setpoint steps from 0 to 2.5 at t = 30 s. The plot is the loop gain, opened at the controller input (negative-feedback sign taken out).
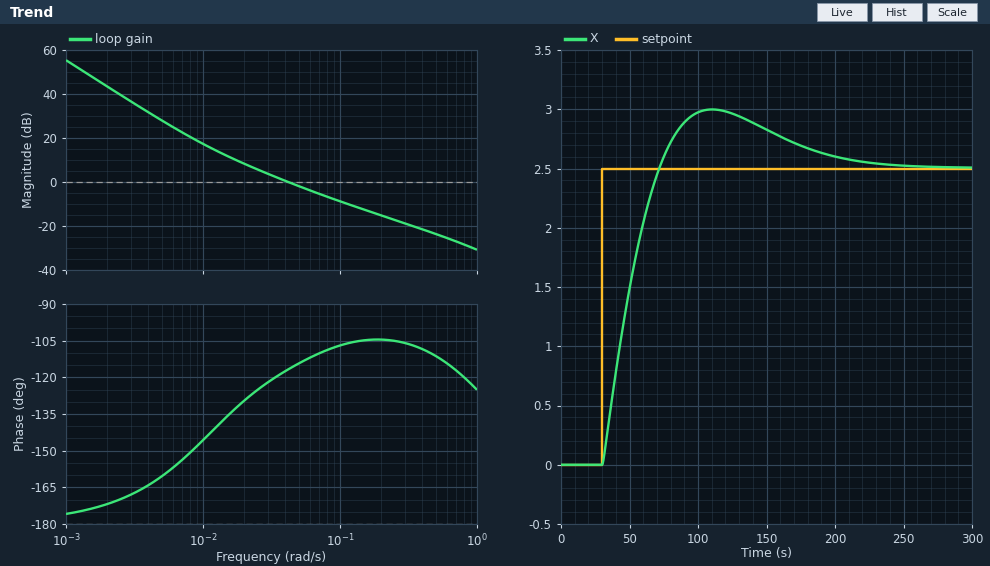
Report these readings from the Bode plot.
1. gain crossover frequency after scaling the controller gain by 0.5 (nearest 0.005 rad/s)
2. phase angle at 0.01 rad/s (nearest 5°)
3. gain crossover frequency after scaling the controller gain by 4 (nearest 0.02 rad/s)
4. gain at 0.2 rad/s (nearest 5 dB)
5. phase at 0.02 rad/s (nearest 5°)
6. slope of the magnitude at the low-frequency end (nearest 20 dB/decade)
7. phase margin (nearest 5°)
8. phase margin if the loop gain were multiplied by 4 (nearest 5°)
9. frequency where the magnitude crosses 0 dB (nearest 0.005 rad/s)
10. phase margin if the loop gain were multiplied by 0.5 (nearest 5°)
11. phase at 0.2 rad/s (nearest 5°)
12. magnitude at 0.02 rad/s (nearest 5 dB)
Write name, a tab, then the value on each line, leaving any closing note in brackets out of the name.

gain crossover frequency after scaling the controller gain by 0.5	0.025 rad/s
phase angle at 0.01 rad/s	-145°
gain crossover frequency after scaling the controller gain by 4	0.14 rad/s
gain at 0.2 rad/s	-15 dB
phase at 0.02 rad/s	-130°
slope of the magnitude at the low-frequency end	-40 dB/decade
phase margin	65°
phase margin if the loop gain were multiplied by 4	75°
frequency where the magnitude crosses 0 dB	0.040 rad/s
phase margin if the loop gain were multiplied by 0.5	55°
phase at 0.2 rad/s	-105°
magnitude at 0.02 rad/s	10 dB
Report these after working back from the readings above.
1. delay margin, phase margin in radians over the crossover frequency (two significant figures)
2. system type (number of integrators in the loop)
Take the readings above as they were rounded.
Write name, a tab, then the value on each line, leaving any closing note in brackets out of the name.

delay margin, phase margin in radians over the crossover frequency	28 s
system type	2
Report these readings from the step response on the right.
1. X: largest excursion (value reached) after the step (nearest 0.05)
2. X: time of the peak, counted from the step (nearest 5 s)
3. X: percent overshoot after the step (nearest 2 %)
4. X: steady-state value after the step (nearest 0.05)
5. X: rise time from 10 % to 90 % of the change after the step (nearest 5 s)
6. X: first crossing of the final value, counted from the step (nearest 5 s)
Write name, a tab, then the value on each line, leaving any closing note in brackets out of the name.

X: largest excursion (value reached) after the step	3.00
X: time of the peak, counted from the step	80 s
X: percent overshoot after the step	20 %
X: steady-state value after the step	2.50
X: rise time from 10 % to 90 % of the change after the step	30 s
X: first crossing of the final value, counted from the step	40 s
